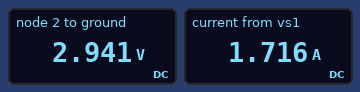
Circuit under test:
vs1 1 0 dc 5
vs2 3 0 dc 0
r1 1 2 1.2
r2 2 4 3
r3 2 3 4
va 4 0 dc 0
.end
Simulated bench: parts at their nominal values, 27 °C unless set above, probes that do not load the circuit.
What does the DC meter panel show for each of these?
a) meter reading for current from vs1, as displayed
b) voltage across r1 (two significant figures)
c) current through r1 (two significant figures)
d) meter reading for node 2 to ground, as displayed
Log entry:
1.716 A
2.1 V
1.7 A
2.941 V
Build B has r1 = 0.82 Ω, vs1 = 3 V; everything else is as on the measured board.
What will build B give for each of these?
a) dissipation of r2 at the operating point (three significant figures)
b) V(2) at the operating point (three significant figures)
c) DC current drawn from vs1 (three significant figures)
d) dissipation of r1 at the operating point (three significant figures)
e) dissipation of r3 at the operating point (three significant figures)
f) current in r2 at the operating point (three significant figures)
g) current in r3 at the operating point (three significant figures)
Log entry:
1.37 W
2.03 V
1.18 A
1.15 W
1.03 W
676 mA
507 mA
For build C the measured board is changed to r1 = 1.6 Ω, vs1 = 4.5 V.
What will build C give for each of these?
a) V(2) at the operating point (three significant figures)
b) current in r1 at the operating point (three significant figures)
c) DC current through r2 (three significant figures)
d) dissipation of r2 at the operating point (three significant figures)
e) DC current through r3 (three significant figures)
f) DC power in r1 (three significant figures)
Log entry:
2.33 V
1.36 A
776 mA
1.81 W
582 mA
2.95 W
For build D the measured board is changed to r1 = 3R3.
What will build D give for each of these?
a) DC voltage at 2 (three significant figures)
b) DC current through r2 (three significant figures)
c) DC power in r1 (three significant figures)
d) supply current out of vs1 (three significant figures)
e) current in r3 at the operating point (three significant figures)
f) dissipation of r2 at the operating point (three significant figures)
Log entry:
1.71 V
570 mA
3.28 W
997 mA
427 mA
974 mW
